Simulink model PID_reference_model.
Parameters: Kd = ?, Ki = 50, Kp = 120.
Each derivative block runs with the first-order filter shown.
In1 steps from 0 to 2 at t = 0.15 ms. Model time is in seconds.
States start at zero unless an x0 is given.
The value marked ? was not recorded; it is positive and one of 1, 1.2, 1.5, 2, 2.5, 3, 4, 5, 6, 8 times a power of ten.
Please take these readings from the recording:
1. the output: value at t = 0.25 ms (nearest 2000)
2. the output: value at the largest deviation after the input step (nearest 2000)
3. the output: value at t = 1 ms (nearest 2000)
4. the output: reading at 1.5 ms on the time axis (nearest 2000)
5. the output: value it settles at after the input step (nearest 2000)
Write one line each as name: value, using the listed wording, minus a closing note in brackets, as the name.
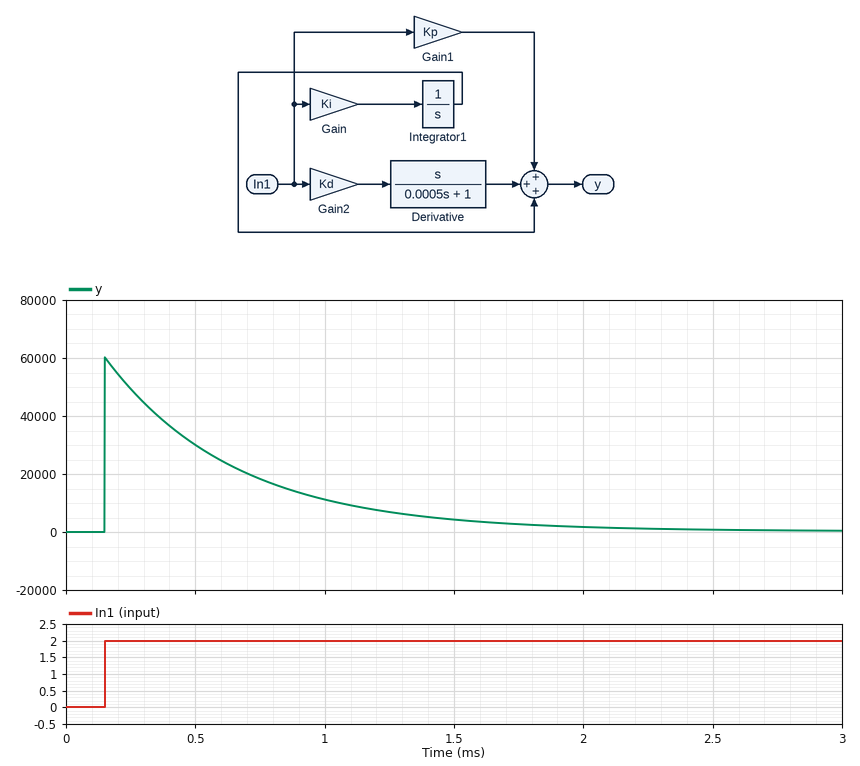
the output: value at t = 0.25 ms: 50000
the output: value at the largest deviation after the input step: 60000
the output: value at t = 1 ms: 12000
the output: reading at 1.5 ms on the time axis: 4000
the output: value it settles at after the input step: 0
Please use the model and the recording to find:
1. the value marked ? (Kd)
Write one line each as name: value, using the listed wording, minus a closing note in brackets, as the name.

the value marked ?: 15
